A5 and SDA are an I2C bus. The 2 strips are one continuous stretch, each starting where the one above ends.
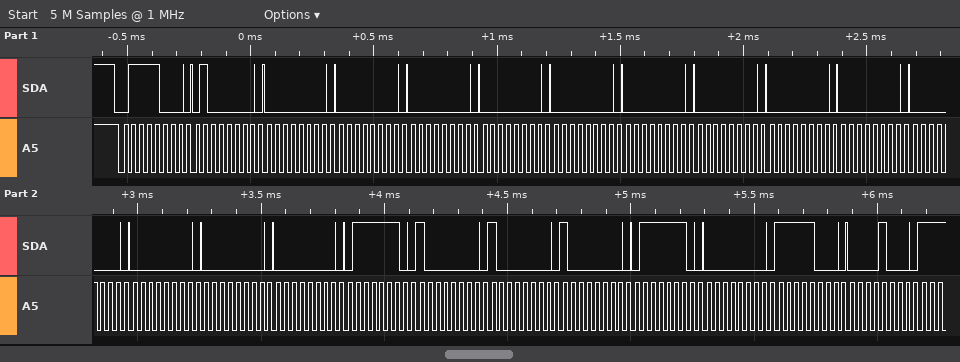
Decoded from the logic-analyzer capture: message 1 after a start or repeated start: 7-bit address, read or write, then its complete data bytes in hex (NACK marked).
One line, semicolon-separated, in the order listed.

0x3C write: 40 00 00 00 00 00 00 00 00 00 00 00 00 00 7E 80 80 80 7E 00 F8 08
